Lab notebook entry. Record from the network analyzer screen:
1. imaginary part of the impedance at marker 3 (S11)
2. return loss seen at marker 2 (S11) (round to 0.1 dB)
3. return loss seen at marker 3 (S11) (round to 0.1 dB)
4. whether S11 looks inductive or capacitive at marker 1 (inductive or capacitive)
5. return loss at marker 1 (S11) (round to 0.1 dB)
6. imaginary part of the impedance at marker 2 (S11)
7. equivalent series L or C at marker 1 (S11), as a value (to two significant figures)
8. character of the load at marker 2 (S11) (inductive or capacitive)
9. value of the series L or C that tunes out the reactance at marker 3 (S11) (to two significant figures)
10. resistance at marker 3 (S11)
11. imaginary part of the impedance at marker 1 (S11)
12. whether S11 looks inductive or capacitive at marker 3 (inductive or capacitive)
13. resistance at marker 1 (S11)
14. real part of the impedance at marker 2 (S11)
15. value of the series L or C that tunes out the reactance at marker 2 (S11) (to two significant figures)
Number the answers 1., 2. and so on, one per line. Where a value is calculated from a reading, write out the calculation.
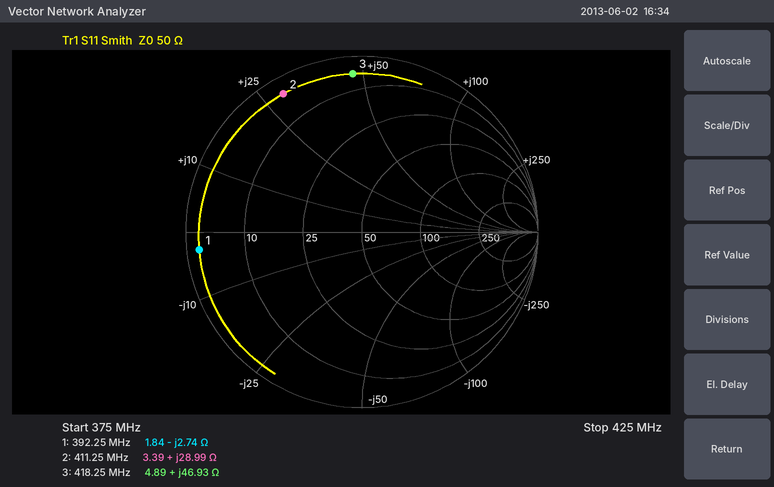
1. +46.93 Ω
2. 0.9 dB
3. 0.9 dB
4. capacitive
5. 0.6 dB
6. +28.99 Ω
7. C = 1/(2π × 392.25 MHz × 2.74 Ω) ≈ 148 pF, so 150 pF to two significant figures
8. inductive
9. C = 1/(2π × 418.25 MHz × 46.93 Ω) ≈ 8.1 pF
10. 4.89 Ω
11. -2.74 Ω
12. inductive
13. 1.84 Ω
14. 3.39 Ω
15. C = 1/(2π × 411.25 MHz × 28.99 Ω) ≈ 13 pF
